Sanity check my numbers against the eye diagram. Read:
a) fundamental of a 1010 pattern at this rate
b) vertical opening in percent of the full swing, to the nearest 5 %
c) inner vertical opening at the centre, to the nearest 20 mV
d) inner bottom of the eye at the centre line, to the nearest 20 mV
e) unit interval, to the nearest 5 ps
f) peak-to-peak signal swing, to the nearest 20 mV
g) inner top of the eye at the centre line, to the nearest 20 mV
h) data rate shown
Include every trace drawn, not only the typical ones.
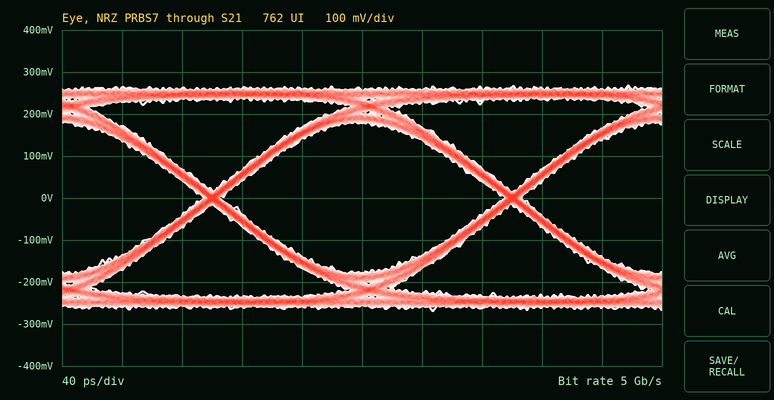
2.5 GHz
65 %
360 mV
-180 mV
200 ps
540 mV
180 mV
5 Gb/s
